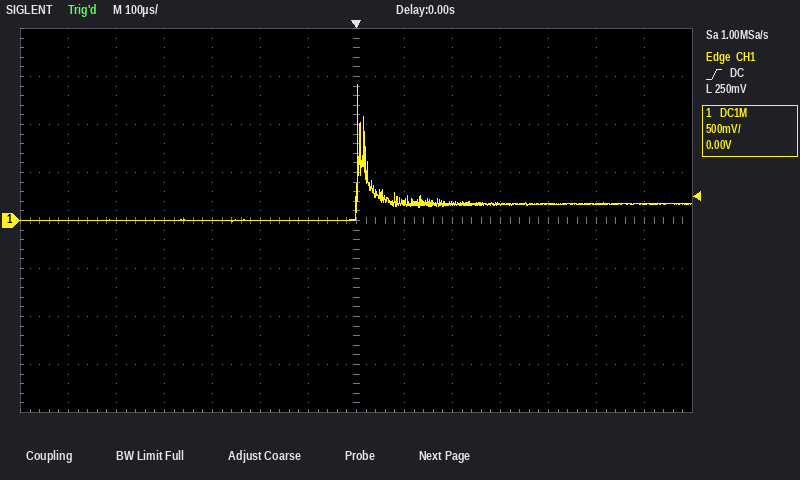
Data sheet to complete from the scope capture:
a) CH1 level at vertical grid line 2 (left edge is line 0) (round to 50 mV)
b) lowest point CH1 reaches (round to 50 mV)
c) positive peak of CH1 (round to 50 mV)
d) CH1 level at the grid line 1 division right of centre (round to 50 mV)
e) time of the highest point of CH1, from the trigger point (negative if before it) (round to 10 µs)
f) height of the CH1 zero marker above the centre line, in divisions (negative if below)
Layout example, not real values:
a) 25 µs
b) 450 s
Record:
a) 0 mV
b) 0 mV
c) 1.40 V
d) 200 mV
e) 0 µs
f) 0.0 div
